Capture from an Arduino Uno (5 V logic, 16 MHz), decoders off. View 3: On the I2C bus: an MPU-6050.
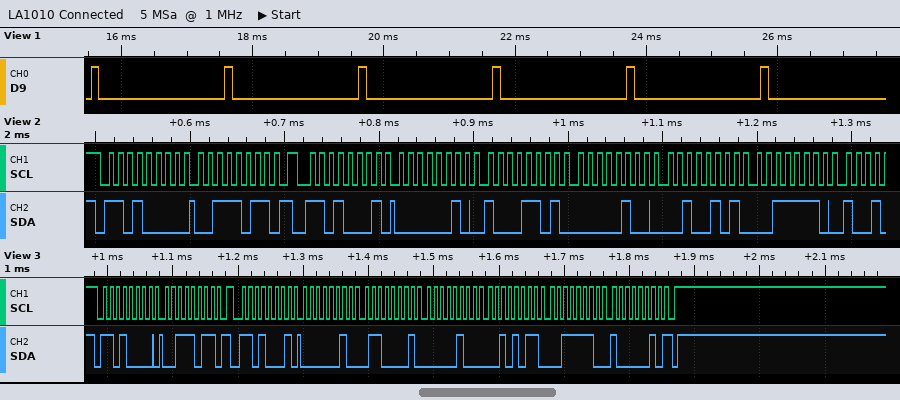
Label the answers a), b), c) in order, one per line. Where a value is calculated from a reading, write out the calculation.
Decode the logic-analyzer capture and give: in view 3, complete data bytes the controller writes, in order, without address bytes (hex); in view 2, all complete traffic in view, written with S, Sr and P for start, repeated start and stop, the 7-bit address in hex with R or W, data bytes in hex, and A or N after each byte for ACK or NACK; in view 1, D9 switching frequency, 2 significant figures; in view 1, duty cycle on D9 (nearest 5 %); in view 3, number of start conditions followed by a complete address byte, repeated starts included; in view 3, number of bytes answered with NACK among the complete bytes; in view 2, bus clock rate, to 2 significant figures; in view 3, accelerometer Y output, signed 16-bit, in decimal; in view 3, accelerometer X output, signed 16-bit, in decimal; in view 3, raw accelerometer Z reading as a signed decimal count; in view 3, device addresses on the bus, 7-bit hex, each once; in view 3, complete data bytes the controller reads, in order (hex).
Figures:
a) 3B
b) S 68W A 3B A Sr 68R A 02 A 8D A 04 A 25 A 3E A
c) 490 Hz
d) 5 %
e) 2
f) 1
g) 100 kHz
h) 0x042B = 1067
i) 0x0261 = 609
j) 0x3E82 = 16002
k) 0x68
l) 02 61 04 2B 3E 82
